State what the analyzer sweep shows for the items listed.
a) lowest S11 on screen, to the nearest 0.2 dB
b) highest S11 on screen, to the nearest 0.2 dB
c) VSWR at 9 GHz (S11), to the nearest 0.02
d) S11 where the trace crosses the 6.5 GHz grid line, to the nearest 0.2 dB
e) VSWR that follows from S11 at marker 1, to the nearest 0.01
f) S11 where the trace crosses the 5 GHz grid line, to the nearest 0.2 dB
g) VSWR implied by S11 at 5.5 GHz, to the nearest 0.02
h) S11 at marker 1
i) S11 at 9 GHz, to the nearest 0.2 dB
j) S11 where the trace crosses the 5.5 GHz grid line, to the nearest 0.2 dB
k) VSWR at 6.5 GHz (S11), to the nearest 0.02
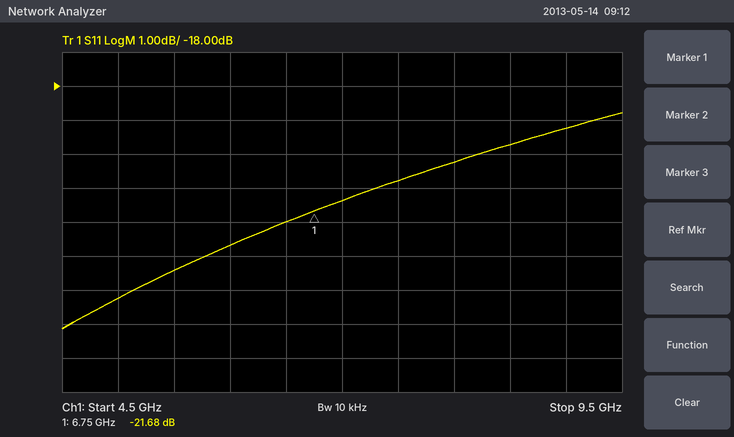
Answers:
-25.2 dB
-18.8 dB
1.24
-22.0 dB
1.18
-24.2 dB
1.14
-21.68 dB
-19.2 dB
-23.4 dB
1.18
